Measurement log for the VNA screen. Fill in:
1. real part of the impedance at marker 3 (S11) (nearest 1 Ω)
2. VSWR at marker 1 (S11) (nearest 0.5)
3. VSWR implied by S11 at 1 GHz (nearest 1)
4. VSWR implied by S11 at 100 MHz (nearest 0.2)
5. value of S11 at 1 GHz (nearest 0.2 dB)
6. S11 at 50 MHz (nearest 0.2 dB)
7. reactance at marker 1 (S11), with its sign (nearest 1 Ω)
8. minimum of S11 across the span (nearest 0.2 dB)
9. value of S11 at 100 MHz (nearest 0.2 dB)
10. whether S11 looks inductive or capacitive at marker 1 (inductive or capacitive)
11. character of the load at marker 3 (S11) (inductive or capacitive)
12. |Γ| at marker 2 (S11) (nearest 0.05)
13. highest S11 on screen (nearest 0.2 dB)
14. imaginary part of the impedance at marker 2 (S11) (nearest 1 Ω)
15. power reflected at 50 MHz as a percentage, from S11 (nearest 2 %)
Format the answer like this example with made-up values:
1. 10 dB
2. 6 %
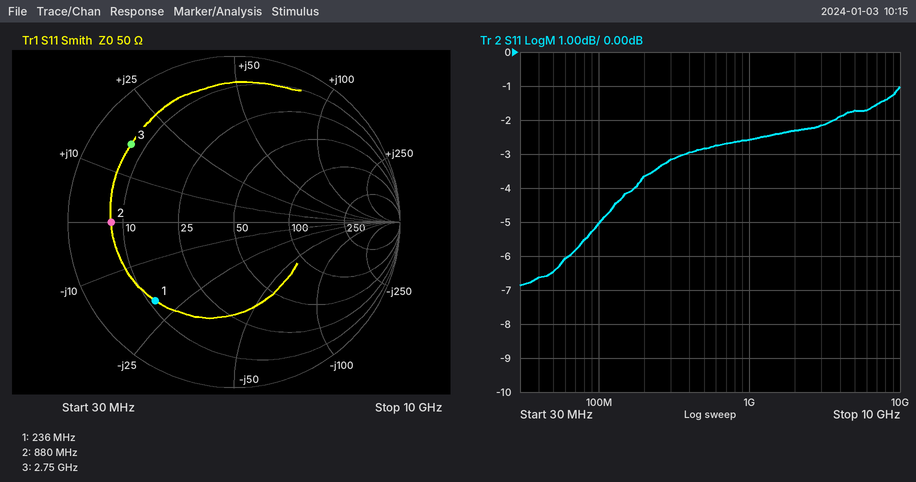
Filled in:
1. 7 Ω
2. 5.0
3. 7
4. 3.6
5. -2.6 dB
6. -6.4 dB
7. -20 Ω
8. -6.8 dB
9. -5.0 dB
10. capacitive
11. inductive
12. 0.75
13. -1.0 dB
14. 0 Ω
15. 22 %
